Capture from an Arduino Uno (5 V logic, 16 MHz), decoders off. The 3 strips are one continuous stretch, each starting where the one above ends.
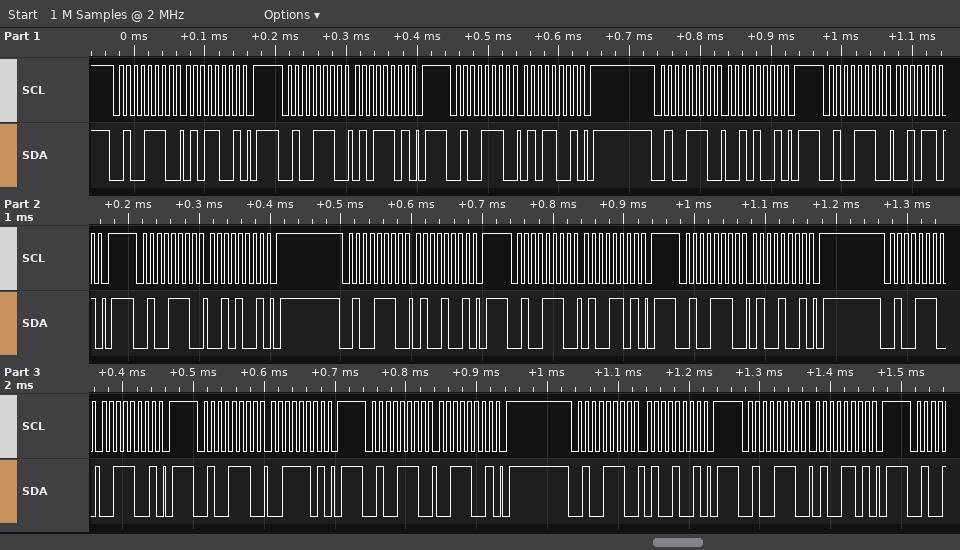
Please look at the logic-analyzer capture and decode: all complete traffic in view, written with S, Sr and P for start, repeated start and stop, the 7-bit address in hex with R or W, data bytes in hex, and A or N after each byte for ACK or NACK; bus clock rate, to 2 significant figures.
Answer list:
S 27W A 59 A P S 27W A 5D A P S 27W A 59 A P S 27W A 29 A P S 27W A 2D A P S 27W A 29 A P S 27W A 49 A P S 27W A 4D A P S 27W A 49 A P S 27W A 39 A P S 27W A 3D A P S 27W A 39 A P S 27W A 49 A P S 27W A 4D A P
100 kHz
